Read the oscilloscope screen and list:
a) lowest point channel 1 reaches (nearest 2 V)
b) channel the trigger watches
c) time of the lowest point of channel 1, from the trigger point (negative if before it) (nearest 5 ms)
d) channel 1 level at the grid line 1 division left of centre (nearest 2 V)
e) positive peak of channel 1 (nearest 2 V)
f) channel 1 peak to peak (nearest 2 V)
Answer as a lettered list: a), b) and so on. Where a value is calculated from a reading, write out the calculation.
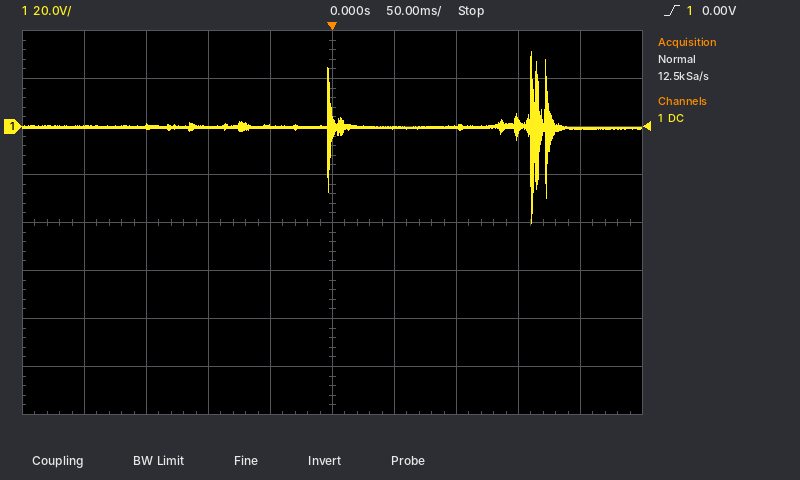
a) -40 V
b) channel 1
c) +160 ms
d) 0 V
e) 32 V
f) 32 V − (-40 V) = 72 V
